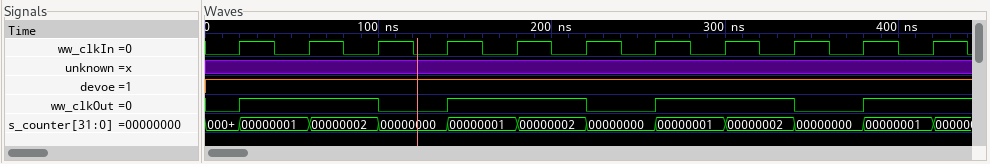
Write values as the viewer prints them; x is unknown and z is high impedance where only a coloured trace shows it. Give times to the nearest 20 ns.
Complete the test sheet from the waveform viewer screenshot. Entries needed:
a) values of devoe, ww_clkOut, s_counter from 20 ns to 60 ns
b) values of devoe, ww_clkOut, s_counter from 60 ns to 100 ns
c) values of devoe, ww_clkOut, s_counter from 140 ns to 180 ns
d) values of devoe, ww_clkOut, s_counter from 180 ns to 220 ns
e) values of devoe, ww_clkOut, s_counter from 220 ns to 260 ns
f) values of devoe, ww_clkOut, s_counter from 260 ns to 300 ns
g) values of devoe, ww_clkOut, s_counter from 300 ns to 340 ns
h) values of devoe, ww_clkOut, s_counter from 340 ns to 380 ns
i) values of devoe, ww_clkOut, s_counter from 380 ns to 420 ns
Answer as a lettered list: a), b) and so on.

a) devoe=1, ww_clkOut=1, s_counter=00000001
b) devoe=1, ww_clkOut=1, s_counter=00000002
c) devoe=1, ww_clkOut=1, s_counter=00000001
d) devoe=1, ww_clkOut=1, s_counter=00000002
e) devoe=1, ww_clkOut=0, s_counter=00000000
f) devoe=1, ww_clkOut=1, s_counter=00000001
g) devoe=1, ww_clkOut=1, s_counter=00000002
h) devoe=1, ww_clkOut=0, s_counter=00000000
i) devoe=1, ww_clkOut=1, s_counter=00000001
